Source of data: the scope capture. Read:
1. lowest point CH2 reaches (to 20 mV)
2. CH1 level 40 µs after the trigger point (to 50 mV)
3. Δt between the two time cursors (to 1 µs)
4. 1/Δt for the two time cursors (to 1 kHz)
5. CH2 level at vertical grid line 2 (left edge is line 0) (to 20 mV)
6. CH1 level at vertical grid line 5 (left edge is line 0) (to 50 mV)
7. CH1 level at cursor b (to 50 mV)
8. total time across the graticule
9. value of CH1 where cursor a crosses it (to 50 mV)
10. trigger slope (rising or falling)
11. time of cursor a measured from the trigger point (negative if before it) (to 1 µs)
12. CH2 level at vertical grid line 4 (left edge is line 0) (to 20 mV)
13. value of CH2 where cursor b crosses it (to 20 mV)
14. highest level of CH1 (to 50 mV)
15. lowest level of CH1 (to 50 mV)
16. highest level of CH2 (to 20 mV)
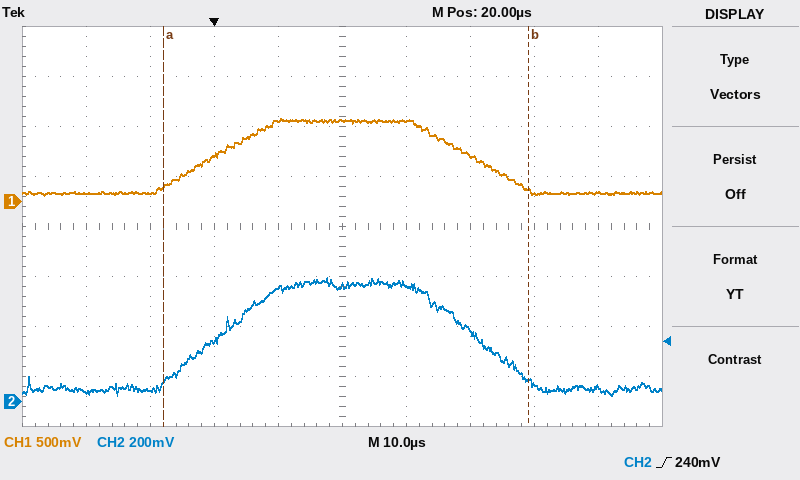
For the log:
20 mV
450 mV
57 µs
18 kHz
40 mV
800 mV
100 mV
100 µs
150 mV
rising
-8 µs
460 mV
80 mV
850 mV
50 mV
500 mV
